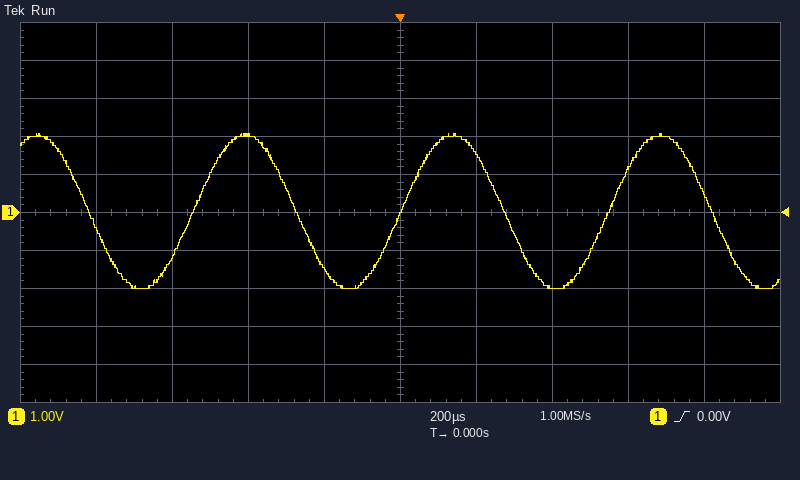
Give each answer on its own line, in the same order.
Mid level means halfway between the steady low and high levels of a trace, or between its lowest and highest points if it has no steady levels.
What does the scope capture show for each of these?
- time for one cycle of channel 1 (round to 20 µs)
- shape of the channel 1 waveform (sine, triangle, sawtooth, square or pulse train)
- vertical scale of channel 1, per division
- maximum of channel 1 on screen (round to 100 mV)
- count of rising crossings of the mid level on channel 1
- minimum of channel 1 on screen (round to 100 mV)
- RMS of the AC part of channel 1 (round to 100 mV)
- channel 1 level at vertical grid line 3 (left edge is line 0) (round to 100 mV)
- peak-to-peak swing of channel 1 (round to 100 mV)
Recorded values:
540 µs
sine
1 V
2.1 V
3
-2.0 V
1.4 V
2.0 V
4.1 V
